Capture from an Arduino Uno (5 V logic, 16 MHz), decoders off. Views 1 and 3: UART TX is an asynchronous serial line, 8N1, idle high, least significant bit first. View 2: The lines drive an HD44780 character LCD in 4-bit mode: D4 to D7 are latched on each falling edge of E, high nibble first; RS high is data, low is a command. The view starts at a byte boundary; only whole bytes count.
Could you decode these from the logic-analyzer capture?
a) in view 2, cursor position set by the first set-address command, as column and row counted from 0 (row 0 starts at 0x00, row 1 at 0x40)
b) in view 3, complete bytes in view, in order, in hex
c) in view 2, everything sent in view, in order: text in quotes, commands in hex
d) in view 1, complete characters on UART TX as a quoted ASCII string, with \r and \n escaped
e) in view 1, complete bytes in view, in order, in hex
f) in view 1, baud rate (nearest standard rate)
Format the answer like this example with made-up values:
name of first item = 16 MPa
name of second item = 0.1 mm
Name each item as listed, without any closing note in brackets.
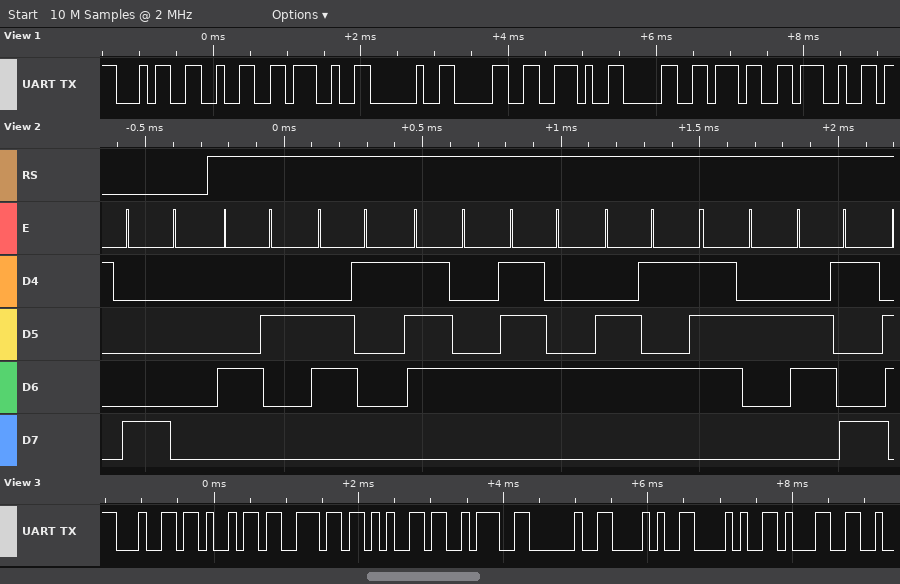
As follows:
in view 2, cursor position set by the first set-address command, as column and row counted from 0 = column 0, row 0
in view 3, complete bytes in view, in order, in hex = 64 69 6E 65 3A 20 28 28 31
in view 2, everything sent in view, in order: text in quotes, commands in hex = 0x80 "Batteri"
in view 1, complete characters on UART TX as a quoted ASCII string, with \r and \n escaped = "42' 0.07'"
in view 1, complete bytes in view, in order, in hex = 34 32 27 20 30 2E 30 37 27
in view 1, baud rate = 9600 baud
